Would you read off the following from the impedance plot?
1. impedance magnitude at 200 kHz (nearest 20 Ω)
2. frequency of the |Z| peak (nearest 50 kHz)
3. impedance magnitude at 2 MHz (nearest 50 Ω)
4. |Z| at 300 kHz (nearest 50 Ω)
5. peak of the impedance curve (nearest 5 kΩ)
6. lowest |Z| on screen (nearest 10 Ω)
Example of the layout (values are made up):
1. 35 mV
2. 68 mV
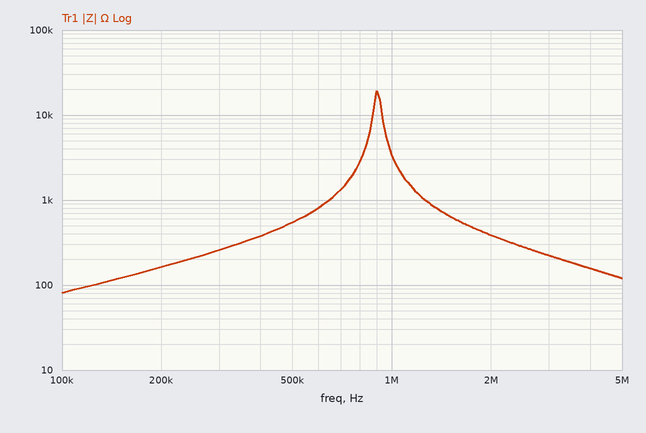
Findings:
1. 160 Ω
2. 900 kHz
3. 400 Ω
4. 250 Ω
5. 20 kΩ
6. 80 Ω
